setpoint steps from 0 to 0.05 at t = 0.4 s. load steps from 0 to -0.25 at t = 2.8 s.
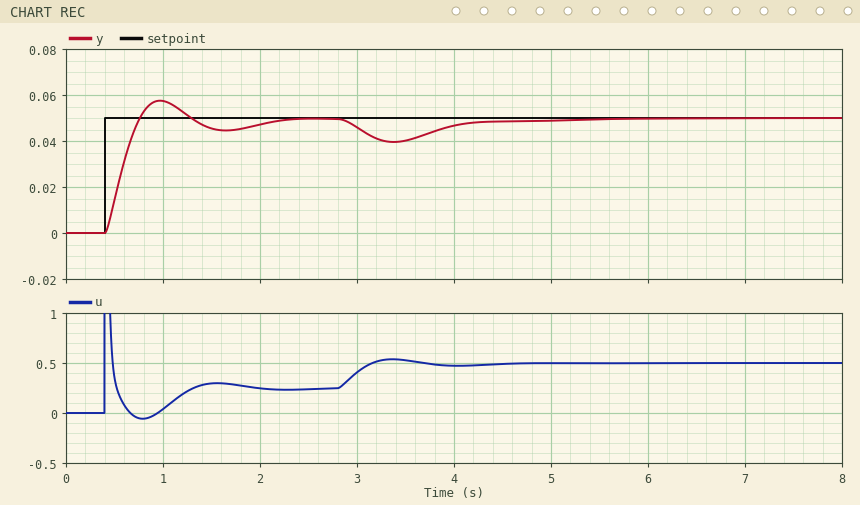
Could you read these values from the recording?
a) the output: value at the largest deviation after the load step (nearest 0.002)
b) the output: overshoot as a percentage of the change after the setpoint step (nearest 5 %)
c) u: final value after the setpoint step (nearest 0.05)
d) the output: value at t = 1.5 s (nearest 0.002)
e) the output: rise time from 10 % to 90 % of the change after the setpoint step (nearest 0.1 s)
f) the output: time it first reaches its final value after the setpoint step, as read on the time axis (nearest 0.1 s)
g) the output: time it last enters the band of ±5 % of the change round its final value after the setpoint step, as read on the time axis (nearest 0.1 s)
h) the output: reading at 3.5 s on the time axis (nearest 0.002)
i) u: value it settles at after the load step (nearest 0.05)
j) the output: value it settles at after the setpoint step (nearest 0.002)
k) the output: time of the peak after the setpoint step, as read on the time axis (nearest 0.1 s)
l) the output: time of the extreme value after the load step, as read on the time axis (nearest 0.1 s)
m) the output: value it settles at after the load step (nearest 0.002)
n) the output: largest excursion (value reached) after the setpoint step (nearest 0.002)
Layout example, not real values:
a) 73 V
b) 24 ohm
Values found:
a) 0.040
b) 15 %
c) 0.25
d) 0.046
e) 0.3 s
f) 0.8 s
g) 2.0 s
h) 0.040
i) 0.50
j) 0.050
k) 1.0 s
l) 3.4 s
m) 0.050
n) 0.058
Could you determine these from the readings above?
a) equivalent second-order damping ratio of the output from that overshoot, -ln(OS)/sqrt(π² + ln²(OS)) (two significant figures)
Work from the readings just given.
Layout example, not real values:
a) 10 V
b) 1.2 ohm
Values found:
a) 0.52
